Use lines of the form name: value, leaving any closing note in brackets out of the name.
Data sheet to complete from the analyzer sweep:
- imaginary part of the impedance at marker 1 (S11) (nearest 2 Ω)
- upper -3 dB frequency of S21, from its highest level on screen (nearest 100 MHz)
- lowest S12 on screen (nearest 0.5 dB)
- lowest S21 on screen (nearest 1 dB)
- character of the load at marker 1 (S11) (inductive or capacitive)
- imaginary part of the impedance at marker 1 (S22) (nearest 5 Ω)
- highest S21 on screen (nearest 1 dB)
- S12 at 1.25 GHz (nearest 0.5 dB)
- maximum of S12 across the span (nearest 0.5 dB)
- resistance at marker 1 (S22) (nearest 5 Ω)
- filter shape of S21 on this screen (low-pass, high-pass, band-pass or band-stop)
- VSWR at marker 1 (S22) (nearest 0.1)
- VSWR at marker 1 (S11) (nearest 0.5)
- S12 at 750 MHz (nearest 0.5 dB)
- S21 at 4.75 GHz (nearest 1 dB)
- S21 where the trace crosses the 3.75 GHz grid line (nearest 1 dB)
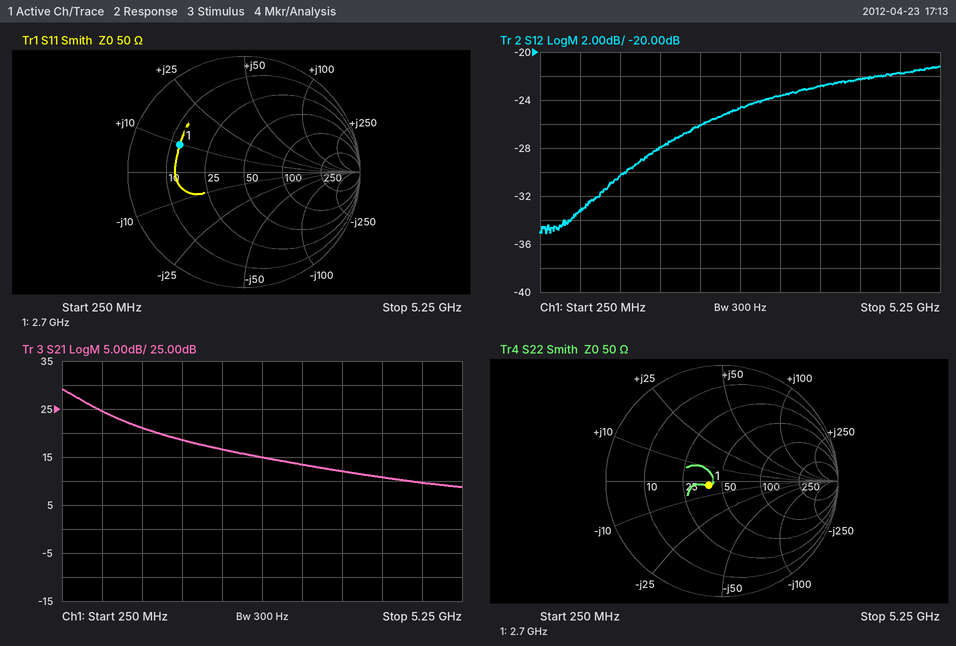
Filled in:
imaginary part of the impedance at marker 1 (S11): +10 Ω
upper -3 dB frequency of S21, from its highest level on screen: 600 MHz
lowest S12 on screen: -35.0 dB
lowest S21 on screen: 9 dB
character of the load at marker 1 (S11): inductive
imaginary part of the impedance at marker 1 (S22): -5 Ω
highest S21 on screen: 29 dB
S12 at 1.25 GHz: -30.5 dB
maximum of S12 across the span: -21.0 dB
resistance at marker 1 (S22): 40 Ω
filter shape of S21 on this screen: low-pass
VSWR at marker 1 (S22): 1.3
VSWR at marker 1 (S11): 4.0
S12 at 750 MHz: -33.0 dB
S21 at 4.75 GHz: 10 dB
S21 where the trace crosses the 3.75 GHz grid line: 12 dB
